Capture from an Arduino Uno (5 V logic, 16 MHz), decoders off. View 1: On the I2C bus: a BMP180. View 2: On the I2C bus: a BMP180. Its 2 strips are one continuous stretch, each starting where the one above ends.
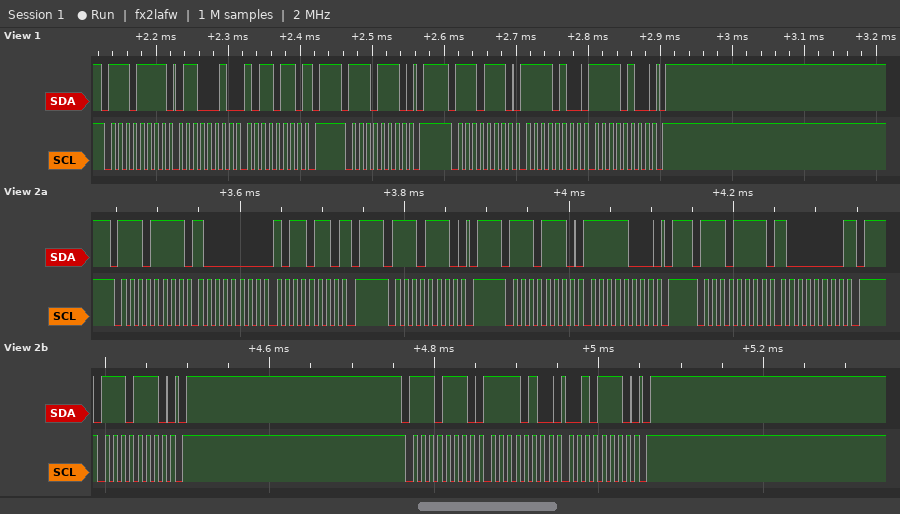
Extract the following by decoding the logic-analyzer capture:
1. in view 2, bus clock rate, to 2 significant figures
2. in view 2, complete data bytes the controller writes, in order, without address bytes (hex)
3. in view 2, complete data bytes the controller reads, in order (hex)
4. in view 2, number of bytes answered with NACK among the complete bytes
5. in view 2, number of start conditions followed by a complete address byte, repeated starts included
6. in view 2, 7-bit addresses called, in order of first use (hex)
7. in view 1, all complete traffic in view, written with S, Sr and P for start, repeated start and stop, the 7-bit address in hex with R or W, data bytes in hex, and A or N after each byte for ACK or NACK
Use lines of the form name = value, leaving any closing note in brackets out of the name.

in view 2, bus clock rate, to 2 significant figures = 100 kHz
in view 2, complete data bytes the controller writes, in order, without address bytes = F8 F4 2E
in view 2, complete data bytes the controller reads, in order = 80 B6 80
in view 2, number of bytes answered with NACK among the complete bytes = 2
in view 2, number of start conditions followed by a complete address byte, repeated starts included = 6
in view 2, 7-bit addresses called, in order of first use = 0x77
in view 1, all complete traffic in view, written with S, Sr and P for start, repeated start and stop, the 7-bit address in hex with R or W, data bytes in hex, and A or N after each byte for ACK or NACK = S 77R A 62 A B6 N P S 77W A P S 77W A F4 A F4 A P
